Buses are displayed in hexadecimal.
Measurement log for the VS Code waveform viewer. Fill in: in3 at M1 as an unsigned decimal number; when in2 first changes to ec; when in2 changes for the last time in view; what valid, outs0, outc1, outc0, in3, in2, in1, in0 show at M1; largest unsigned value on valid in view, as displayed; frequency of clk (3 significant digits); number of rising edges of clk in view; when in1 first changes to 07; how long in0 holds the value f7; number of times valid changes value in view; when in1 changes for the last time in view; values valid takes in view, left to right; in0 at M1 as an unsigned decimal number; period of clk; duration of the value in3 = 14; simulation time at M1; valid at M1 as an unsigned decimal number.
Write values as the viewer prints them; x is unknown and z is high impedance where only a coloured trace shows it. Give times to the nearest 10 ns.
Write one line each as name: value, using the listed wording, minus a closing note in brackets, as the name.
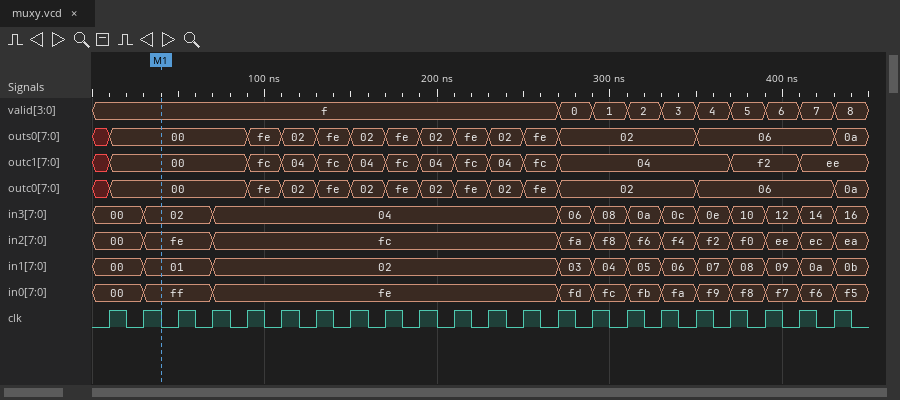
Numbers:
in3 at M1 as an unsigned decimal number: 2
when in2 first changes to ec: 410 ns
when in2 changes for the last time in view: 430 ns
what valid, outs0, outc1, outc0, in3, in2, in1, in0 show at M1: valid=f, outs0=00, outc1=00, outc0=00, in3=02, in2=fe, in1=01, in0=ff
largest unsigned value on valid in view, as displayed: f
frequency of clk: 50.0 MHz
number of rising edges of clk in view: 22
when in1 first changes to 07: 350 ns
how long in0 holds the value f7: 20 ns
number of times valid changes value in view: 9
when in1 changes for the last time in view: 430 ns
values valid takes in view, left to right: f, 0, 1, 2, 3, 4, 5, 6, 7, 8
in0 at M1 as an unsigned decimal number: 255
period of clk: 20 ns
duration of the value in3 = 14: 20 ns
simulation time at M1: 40 ns
valid at M1 as an unsigned decimal number: 15
